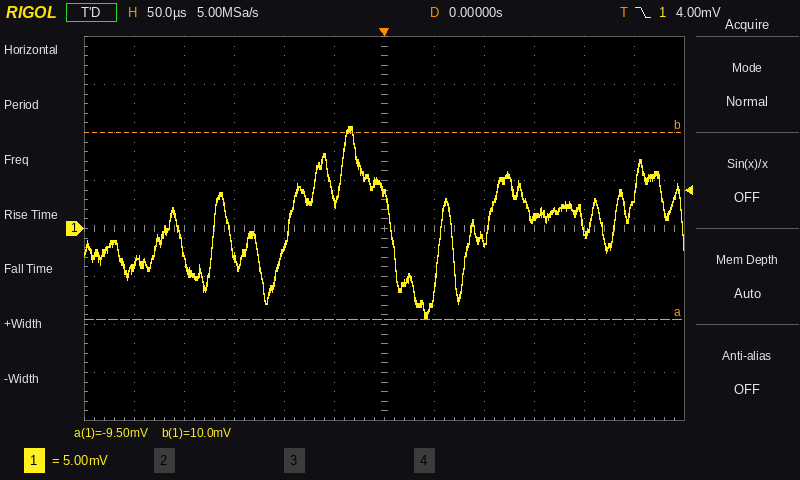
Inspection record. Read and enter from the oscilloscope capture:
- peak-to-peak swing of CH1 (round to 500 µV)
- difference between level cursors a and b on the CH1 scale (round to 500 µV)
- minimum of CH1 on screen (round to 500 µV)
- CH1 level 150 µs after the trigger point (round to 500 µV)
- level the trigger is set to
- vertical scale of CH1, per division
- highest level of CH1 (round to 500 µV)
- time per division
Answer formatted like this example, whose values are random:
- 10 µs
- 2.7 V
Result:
- 20.0 mV
- 19.5 mV
- -9.5 mV
- 1.0 mV
- 4.00 mV
- 5 mV
- 10.5 mV
- 50 µs
